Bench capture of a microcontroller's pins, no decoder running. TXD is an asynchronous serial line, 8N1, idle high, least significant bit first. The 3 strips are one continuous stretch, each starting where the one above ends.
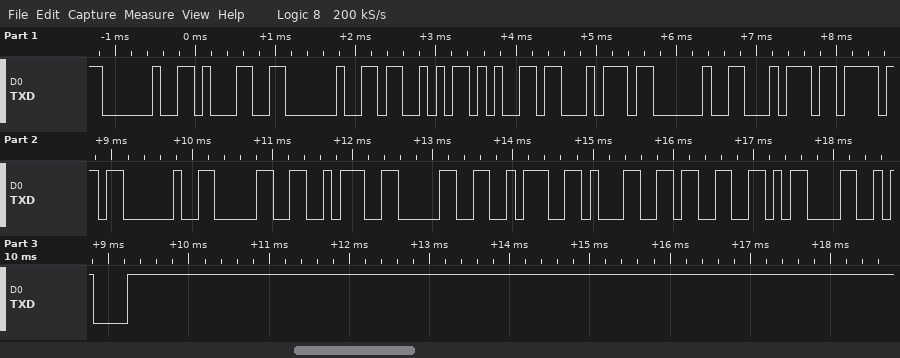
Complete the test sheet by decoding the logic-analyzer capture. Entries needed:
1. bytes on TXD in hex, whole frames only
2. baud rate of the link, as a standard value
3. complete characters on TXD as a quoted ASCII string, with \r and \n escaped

20 31 20 53 65 74 20 74 6F 20 30 3A 30 3A 31 33 0D 0A
9600 baud
" 1 Set to 0:0:13\r\n"
